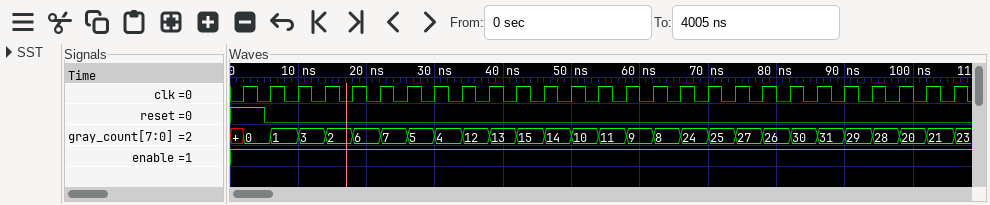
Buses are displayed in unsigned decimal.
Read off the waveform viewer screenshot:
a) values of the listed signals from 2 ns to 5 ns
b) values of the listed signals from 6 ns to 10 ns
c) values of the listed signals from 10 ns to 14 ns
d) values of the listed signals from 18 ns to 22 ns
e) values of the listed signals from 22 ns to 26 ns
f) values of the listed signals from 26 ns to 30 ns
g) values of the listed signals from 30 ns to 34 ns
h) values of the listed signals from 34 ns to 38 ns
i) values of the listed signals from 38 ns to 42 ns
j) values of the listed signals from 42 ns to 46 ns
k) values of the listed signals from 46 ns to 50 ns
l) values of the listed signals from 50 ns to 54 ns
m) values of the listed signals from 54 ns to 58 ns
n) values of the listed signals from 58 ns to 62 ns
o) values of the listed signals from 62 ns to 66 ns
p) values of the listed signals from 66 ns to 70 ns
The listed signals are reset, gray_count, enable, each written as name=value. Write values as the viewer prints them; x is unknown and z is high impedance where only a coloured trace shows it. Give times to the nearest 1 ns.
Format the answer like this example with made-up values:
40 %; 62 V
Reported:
reset=1, gray_count=0, enable=1; reset=0, gray_count=1, enable=1; reset=0, gray_count=3, enable=1; reset=0, gray_count=6, enable=1; reset=0, gray_count=7, enable=1; reset=0, gray_count=5, enable=1; reset=0, gray_count=4, enable=1; reset=0, gray_count=12, enable=1; reset=0, gray_count=13, enable=1; reset=0, gray_count=15, enable=1; reset=0, gray_count=14, enable=1; reset=0, gray_count=10, enable=1; reset=0, gray_count=11, enable=1; reset=0, gray_count=9, enable=1; reset=0, gray_count=8, enable=1; reset=0, gray_count=24, enable=1
